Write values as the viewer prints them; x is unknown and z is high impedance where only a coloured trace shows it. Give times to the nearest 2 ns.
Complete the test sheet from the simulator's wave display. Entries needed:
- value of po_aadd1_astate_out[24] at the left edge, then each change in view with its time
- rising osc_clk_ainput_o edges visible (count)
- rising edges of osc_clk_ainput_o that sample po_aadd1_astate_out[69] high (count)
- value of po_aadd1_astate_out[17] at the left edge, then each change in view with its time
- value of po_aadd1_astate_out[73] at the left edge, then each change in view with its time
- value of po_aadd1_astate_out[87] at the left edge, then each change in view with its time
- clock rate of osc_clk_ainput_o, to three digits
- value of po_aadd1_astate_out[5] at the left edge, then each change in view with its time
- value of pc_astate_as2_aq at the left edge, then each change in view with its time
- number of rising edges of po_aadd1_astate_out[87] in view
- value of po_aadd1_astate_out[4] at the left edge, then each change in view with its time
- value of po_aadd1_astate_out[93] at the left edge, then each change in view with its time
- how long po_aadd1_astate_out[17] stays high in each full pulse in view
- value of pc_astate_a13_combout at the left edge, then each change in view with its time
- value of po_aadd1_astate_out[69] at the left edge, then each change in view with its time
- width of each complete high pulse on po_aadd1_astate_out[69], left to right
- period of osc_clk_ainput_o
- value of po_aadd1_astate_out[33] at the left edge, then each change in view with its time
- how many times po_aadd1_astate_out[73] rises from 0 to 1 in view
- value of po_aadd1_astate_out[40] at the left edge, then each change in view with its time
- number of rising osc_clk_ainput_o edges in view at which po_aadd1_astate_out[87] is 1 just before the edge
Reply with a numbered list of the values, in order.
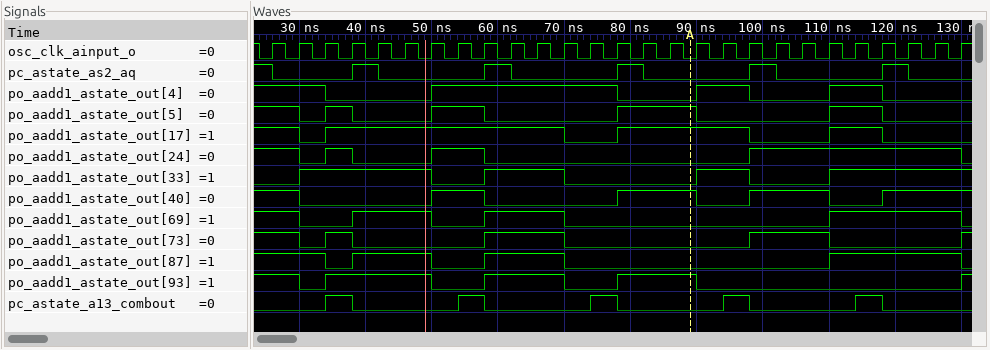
1. 1, 0 at 30 ns, 1 at 34 ns, 0 at 38 ns, 1 at 50 ns, 0 at 58 ns, 1 at 98 ns, 0 at 130 ns
2. 27
3. 13
4. 1, 0 at 30 ns, 1 at 34 ns, 0 at 70 ns, 1 at 78 ns, 0 at 98 ns, 1 at 110 ns, 0 at 118 ns
5. 1, 0 at 30 ns, 1 at 34 ns, 0 at 38 ns, 1 at 58 ns, 0 at 70 ns, 1 at 98 ns, 0 at 110 ns, 1 at 130 ns
6. 1, 0 at 34 ns, 1 at 38 ns, 0 at 50 ns, 1 at 58 ns, 0 at 70 ns, 1 at 110 ns, 0 at 130 ns
7. 250 MHz
8. 1, 0 at 30 ns, 1 at 34 ns, 0 at 38 ns, 1 at 50 ns, 0 at 58 ns, 1 at 78 ns, 0 at 90 ns, 1 at 110 ns, 0 at 118 ns
9. 1, 0 at 26 ns, 1 at 38 ns, 0 at 42 ns, 1 at 58 ns, 0 at 62 ns, 1 at 78 ns, 0 at 82 ns, 1 at 98 ns, 0 at 102 ns, 1 at 118 ns, 0 at 122 ns
10. 3
11. 1, 0 at 34 ns, 1 at 50 ns, 0 at 78 ns, 1 at 90 ns, 0 at 98 ns, 1 at 110 ns, 0 at 118 ns
12. 1, 0 at 30 ns, 1 at 34 ns, 0 at 50 ns, 1 at 58 ns, 0 at 70 ns, 1 at 78 ns, 0 at 90 ns, 1 at 130 ns
13. 36 ns, 20 ns, 8 ns
14. 0, 1 at 34 ns, 0 at 38 ns, 1 at 54 ns, 0 at 58 ns, 1 at 74 ns, 0 at 78 ns, 1 at 94 ns, 0 at 98 ns, 1 at 114 ns, 0 at 118 ns
15. 1, 0 at 30 ns, 1 at 38 ns, 0 at 50 ns, 1 at 58 ns, 0 at 70 ns, 1 at 110 ns, 0 at 130 ns
16. 12 ns, 12 ns, 20 ns
17. 4 ns
18. 0, 1 at 30 ns, 0 at 50 ns, 1 at 58 ns, 0 at 70 ns, 1 at 90 ns, 0 at 98 ns, 1 at 110 ns
19. 4
20. 1, 0 at 30 ns, 1 at 50 ns, 0 at 58 ns, 1 at 78 ns, 0 at 90 ns, 1 at 98 ns, 0 at 110 ns, 1 at 118 ns
21. 14
